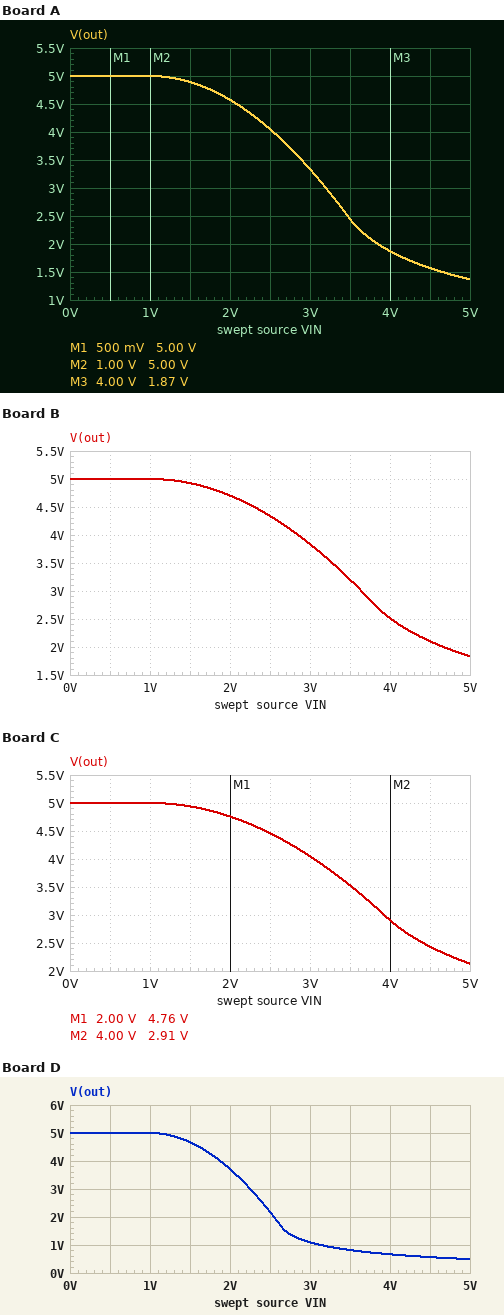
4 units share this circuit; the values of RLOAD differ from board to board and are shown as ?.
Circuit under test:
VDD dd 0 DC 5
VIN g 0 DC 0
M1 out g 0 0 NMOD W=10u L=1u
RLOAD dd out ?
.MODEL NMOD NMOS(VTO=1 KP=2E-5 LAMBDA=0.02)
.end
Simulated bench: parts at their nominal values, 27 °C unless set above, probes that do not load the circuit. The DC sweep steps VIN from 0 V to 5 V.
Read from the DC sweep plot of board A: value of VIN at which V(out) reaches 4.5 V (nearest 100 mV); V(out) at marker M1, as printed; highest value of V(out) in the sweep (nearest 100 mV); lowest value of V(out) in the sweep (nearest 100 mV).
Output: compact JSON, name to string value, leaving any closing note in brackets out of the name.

{"value of VIN at which V(out) reaches 4.5 V": "2.1 V", "V(out) at marker M1, as printed": "5.00 V", "highest value of V(out) in the sweep": "5.0 V", "lowest value of V(out) in the sweep": "1.4 V"}
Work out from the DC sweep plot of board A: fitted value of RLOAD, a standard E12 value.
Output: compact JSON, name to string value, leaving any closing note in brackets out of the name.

{"fitted value of RLOAD, a standard E12 value": "3.9 kΩ"}
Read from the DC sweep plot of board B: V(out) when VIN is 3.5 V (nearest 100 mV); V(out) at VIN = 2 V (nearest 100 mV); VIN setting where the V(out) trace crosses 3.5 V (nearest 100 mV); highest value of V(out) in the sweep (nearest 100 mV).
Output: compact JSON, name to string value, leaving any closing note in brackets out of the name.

{"V(out) when VIN is 3.5 V": "3.2 V", "V(out) at VIN = 2 V": "4.7 V", "VIN setting where the V(out) trace crosses 3.5 V": "3.3 V", "highest value of V(out) in the sweep": "5.0 V"}
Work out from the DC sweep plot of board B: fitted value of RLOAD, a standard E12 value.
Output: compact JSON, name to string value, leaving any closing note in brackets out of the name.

{"fitted value of RLOAD, a standard E12 value": "2.7 kΩ"}
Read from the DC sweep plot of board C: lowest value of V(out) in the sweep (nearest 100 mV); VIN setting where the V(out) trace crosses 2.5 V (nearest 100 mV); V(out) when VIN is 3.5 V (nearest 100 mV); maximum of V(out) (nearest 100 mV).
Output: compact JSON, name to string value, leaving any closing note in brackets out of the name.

{"lowest value of V(out) in the sweep": "2.1 V", "VIN setting where the V(out) trace crosses 2.5 V": "4.4 V", "V(out) when VIN is 3.5 V": "3.5 V", "maximum of V(out)": "5.0 V"}
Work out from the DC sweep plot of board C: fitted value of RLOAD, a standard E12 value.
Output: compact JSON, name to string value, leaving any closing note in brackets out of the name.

{"fitted value of RLOAD, a standard E12 value": "2.2 kΩ"}
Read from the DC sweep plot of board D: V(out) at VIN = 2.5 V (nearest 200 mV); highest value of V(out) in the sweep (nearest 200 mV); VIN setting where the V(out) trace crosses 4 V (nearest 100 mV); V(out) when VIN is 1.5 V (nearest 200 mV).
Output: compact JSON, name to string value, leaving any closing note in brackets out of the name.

{"V(out) at VIN = 2.5 V": "2.2 V", "highest value of V(out) in the sweep": "5.0 V", "VIN setting where the V(out) trace crosses 4 V": "1.9 V", "V(out) when VIN is 1.5 V": "4.6 V"}
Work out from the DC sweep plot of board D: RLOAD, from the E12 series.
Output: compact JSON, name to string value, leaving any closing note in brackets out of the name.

{"RLOAD, from the E12 series": "12 kΩ"}
